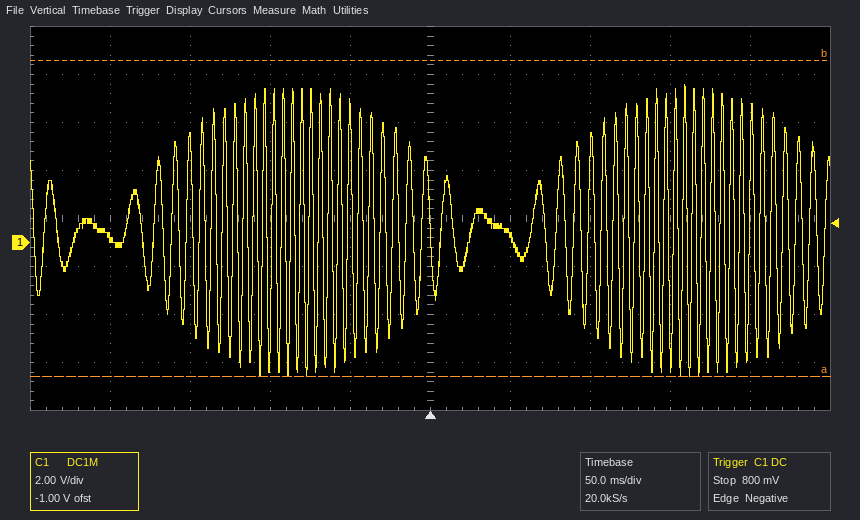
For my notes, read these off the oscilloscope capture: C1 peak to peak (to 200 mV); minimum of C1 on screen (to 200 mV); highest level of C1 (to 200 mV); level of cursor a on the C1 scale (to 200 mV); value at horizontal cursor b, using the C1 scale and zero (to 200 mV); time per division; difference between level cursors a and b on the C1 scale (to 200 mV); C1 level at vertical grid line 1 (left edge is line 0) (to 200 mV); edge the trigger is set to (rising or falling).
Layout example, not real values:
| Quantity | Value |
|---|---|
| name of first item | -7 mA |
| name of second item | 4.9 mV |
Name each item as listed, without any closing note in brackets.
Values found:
| Quantity | Value |
|---|---|
| C1 peak to peak | 12.2 V |
| minimum of C1 on screen | -5.6 V |
| highest level of C1 | 6.6 V |
| level of cursor a on the C1 scale | -5.6 V |
| value at horizontal cursor b, using the C1 scale and zero | 7.6 V |
| time per division | 50 ms |
| difference between level cursors a and b on the C1 scale | 13.2 V |
| C1 level at vertical grid line 1 (left edge is line 0) | 200 mV |
| edge the trigger is set to | falling |
